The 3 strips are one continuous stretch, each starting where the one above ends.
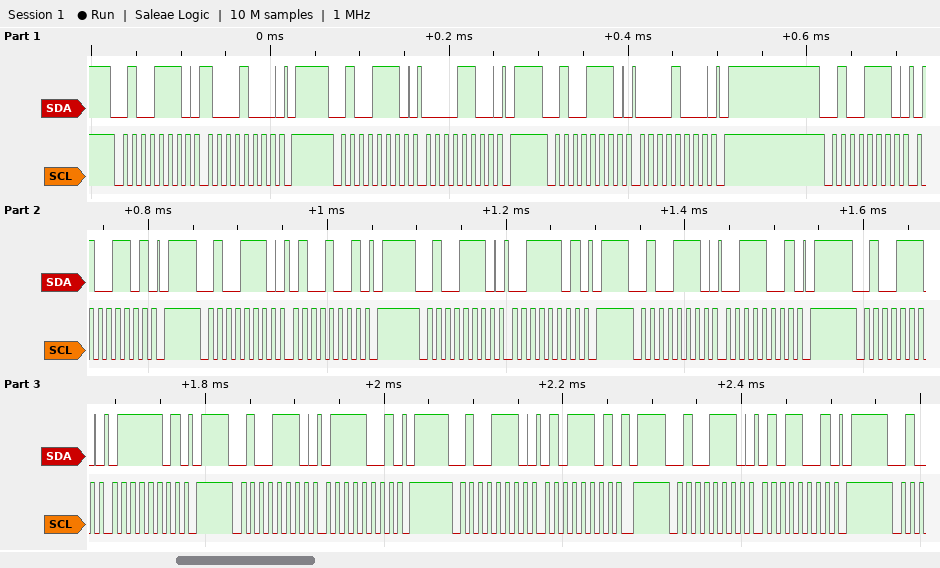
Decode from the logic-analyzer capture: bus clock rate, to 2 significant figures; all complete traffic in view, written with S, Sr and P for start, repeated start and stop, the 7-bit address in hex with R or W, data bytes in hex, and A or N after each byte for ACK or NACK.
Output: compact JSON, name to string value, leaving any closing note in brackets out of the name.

{"bus clock rate, to 2 significant figures": "100 kHz", "all complete traffic in view, written with S, Sr and P for start, repeated start and stop, the 7-bit address in hex with R or W, data bytes in hex, and A or N after each byte for ACK or NACK": "S 27W A 88 A P S 27W A 0C A P S 27W A 08 A P S 27W A 4D A P S 27W A 49 A P S 27W A 3D A P S 27W A 39 A P S 27W A 7D A P S 27W A 79 A P S 27W A 5D A P S 27W A 59 A P"}
